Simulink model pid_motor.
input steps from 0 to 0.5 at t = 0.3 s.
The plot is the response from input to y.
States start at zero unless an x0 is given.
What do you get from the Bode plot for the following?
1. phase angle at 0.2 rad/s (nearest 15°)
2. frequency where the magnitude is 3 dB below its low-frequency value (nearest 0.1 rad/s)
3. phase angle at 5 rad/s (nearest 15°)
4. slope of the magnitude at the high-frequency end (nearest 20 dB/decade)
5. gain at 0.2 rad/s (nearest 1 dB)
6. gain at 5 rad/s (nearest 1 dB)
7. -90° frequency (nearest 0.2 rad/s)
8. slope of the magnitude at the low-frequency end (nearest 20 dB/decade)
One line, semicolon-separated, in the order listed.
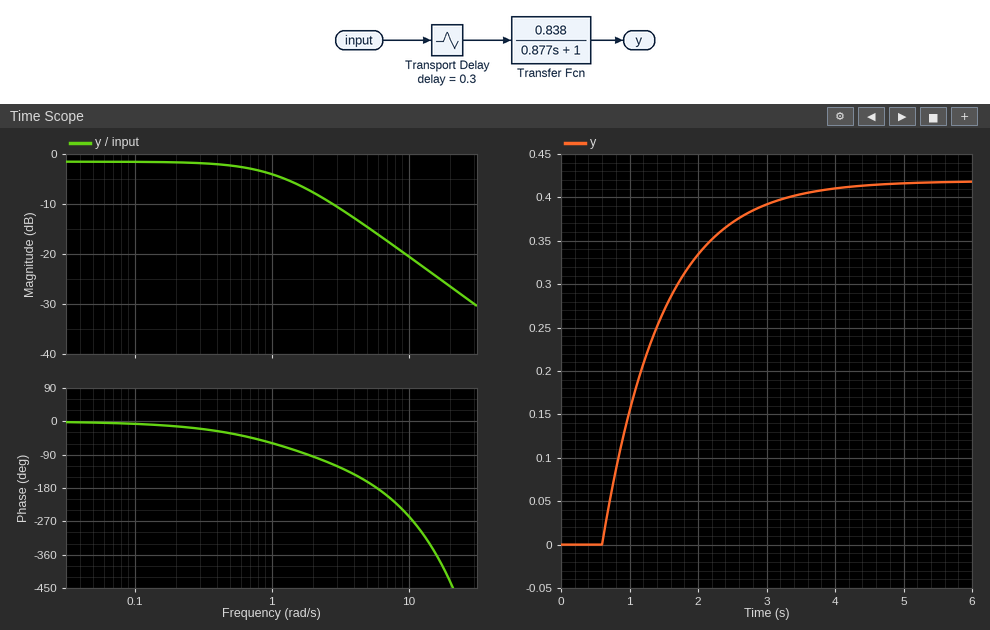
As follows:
-15°; 1.1 rad/s; -165°; -20 dB/decade; -2 dB; -15 dB; 1.8 rad/s; 0 dB/decade
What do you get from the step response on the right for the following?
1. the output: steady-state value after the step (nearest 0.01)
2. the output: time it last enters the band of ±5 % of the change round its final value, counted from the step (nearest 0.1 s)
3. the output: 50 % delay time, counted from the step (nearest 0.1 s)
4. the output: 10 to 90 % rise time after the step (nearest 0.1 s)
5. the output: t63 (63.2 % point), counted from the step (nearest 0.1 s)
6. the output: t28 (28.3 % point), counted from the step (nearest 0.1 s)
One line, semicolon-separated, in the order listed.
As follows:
0.42; 2.9 s; 0.9 s; 1.9 s; 1.2 s; 0.6 s
